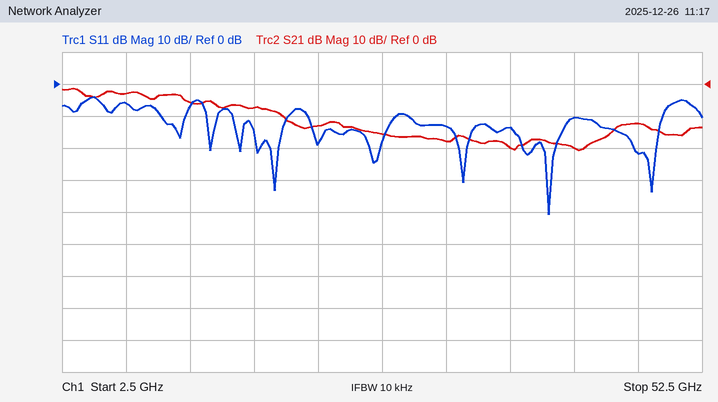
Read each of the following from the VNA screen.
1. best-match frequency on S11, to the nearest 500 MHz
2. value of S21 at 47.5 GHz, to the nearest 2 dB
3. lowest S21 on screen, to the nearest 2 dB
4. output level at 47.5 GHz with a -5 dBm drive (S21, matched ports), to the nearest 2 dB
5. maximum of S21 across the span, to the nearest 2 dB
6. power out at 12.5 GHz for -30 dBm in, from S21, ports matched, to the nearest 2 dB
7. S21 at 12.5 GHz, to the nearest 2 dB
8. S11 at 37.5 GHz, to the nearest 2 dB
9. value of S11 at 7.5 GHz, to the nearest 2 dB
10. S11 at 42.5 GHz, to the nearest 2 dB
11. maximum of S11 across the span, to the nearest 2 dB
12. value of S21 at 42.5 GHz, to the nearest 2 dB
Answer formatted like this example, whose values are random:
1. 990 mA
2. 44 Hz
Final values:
1. 40.5 GHz
2. -12 dB
3. -20 dB
4. -18 dBm
5. -2 dB
6. -36 dBm
7. -6 dB
8. -14 dB
9. -6 dB
10. -10 dB
11. -4 dB
12. -20 dB
